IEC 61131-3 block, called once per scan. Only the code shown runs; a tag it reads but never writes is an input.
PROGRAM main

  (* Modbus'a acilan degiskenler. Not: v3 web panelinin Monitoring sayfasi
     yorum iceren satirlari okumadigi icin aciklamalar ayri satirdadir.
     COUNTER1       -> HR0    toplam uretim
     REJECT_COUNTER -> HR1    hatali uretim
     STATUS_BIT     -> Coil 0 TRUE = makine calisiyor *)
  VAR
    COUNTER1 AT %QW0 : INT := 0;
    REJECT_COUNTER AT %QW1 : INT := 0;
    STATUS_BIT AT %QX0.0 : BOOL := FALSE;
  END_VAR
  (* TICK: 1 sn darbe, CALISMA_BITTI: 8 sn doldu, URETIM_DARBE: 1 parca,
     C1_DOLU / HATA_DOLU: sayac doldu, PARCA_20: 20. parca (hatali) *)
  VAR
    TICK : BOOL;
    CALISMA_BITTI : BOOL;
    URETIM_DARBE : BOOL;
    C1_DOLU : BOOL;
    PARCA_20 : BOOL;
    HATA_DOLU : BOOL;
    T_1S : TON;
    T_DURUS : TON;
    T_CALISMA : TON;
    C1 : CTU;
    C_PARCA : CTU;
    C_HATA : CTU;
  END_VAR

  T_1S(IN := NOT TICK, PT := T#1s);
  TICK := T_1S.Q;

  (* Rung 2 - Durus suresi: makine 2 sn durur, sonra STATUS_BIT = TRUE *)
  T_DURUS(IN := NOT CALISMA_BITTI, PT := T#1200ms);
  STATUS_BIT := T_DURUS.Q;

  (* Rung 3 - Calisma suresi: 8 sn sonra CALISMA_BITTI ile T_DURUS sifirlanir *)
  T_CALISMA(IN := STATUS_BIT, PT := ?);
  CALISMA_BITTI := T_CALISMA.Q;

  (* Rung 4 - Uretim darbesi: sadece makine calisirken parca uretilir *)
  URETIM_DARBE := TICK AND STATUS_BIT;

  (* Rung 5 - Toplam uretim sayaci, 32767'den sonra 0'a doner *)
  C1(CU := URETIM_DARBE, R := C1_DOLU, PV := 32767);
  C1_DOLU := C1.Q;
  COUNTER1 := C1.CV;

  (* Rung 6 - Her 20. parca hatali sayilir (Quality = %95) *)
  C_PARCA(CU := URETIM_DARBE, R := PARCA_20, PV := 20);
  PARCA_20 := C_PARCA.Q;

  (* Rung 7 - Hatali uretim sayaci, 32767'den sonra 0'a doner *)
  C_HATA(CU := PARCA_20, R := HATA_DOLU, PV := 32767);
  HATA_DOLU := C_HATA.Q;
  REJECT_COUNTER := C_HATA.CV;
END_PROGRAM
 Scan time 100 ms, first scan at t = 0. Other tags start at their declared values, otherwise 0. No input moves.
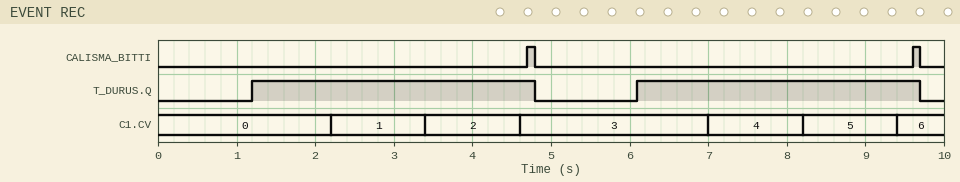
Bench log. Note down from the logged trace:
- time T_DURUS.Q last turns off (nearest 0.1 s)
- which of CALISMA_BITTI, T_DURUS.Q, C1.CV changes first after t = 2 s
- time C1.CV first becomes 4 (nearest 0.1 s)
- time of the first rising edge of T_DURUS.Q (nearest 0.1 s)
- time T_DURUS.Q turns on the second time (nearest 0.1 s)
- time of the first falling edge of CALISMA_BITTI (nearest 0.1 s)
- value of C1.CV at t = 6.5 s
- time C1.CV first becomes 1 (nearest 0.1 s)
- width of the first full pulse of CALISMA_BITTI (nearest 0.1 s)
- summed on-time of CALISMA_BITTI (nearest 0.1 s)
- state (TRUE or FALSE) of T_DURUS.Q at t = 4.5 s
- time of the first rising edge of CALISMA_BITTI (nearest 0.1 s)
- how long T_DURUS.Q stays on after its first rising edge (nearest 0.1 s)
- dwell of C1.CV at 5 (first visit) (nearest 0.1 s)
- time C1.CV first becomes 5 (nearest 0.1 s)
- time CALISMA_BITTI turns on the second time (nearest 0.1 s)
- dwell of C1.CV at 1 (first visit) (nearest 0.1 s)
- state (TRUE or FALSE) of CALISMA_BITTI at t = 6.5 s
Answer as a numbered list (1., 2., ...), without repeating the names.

1. 9.7 s
2. C1.CV
3. 7.0 s
4. 1.2 s
5. 6.1 s
6. 4.8 s
7. 3
8. 2.2 s
9. 0.1 s
10. 0.2 s
11. TRUE
12. 4.7 s
13. 3.6 s
14. 1.2 s
15. 8.2 s
16. 9.6 s
17. 1.2 s
18. FALSE
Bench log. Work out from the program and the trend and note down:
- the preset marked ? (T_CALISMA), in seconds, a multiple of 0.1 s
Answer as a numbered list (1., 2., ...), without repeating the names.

1. 3.5 s
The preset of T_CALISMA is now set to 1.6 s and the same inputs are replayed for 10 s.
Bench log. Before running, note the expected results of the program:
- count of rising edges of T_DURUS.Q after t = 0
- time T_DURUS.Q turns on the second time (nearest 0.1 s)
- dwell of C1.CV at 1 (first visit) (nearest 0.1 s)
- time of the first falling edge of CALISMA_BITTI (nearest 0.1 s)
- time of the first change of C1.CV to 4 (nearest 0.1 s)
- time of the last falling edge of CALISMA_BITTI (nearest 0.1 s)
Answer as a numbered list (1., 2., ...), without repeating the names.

1. 3
2. 4.2 s
3. 2.4 s
4. 2.9 s
5. 8.2 s
6. 8.9 s
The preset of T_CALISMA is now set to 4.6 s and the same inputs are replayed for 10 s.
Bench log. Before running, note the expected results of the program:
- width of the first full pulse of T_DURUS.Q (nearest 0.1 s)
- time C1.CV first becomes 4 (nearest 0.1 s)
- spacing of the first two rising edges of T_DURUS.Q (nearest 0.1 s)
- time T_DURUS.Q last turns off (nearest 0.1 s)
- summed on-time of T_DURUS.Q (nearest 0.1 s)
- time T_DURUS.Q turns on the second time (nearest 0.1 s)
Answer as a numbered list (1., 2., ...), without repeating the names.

1. 4.7 s
2. 5.8 s
3. 6.0 s
4. 5.9 s
5. 7.5 s
6. 7.2 s
